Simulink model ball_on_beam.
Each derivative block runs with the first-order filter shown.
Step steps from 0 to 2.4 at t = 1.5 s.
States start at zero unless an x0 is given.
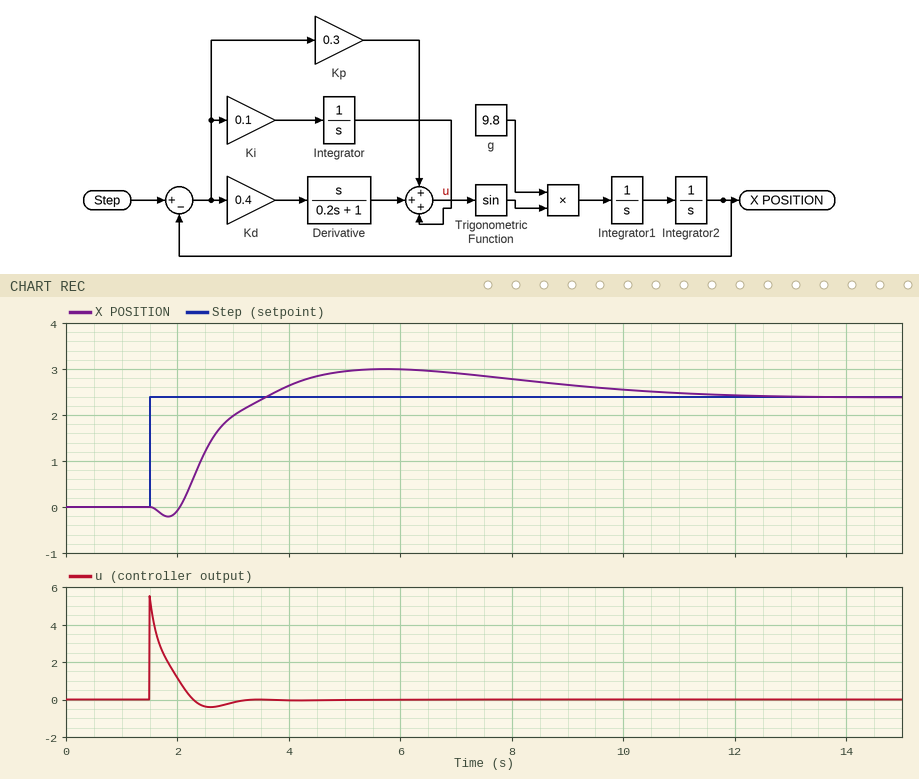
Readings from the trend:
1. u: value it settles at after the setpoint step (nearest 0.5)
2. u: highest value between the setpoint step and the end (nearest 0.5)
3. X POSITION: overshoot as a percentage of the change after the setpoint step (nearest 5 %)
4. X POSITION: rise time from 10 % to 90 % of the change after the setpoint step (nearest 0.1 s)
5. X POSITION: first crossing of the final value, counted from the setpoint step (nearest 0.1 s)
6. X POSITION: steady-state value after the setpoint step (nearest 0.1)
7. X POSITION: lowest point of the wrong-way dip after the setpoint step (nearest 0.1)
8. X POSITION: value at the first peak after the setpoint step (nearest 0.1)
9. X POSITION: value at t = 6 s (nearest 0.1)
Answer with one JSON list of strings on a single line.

["0.0", "5.5", "25 %", "1.1 s", "2.1 s", "2.4", "-0.2", "3.0", "3.0"]
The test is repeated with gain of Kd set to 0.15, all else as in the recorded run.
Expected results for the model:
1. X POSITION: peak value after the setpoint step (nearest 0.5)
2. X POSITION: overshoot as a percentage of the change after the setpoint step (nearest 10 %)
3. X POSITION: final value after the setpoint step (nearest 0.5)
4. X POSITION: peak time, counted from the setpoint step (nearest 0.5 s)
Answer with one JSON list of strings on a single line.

["3.5", "50 %", "2.5", "1.5 s"]
